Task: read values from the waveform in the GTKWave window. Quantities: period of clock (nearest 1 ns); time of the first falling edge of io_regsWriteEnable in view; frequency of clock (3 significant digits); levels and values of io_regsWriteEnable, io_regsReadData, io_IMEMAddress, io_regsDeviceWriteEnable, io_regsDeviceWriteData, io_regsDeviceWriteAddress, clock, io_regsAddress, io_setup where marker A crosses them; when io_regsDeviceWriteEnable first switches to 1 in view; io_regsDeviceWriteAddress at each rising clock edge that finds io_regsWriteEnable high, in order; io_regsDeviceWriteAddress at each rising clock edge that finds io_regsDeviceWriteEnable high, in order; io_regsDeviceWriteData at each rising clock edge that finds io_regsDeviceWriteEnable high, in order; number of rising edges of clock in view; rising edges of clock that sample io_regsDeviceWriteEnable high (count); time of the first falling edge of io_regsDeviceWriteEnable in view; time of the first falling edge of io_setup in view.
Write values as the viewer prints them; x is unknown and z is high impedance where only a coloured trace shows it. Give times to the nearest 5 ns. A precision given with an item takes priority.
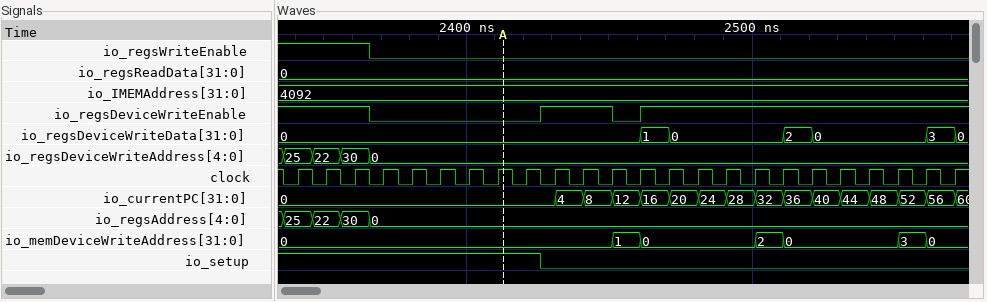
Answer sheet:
10 ns
2365 ns
100 MHz
io_regsWriteEnable=0, io_regsReadData=0, io_IMEMAddress=4092, io_regsDeviceWriteEnable=0, io_regsDeviceWriteData=0, io_regsDeviceWriteAddress=0, clock=1, io_regsAddress=0, io_setup=1
2425 ns
25, 22, 30
25, 22, 30, 0, 0, 0, 0, 0, 0, 0, 0, 0, 0, 0, 0, 0, 0
0, 0, 0, 0, 0, 0, 1, 0, 0, 0, 0, 2, 0, 0, 0, 0, 3
24
17
2365 ns
2425 ns
